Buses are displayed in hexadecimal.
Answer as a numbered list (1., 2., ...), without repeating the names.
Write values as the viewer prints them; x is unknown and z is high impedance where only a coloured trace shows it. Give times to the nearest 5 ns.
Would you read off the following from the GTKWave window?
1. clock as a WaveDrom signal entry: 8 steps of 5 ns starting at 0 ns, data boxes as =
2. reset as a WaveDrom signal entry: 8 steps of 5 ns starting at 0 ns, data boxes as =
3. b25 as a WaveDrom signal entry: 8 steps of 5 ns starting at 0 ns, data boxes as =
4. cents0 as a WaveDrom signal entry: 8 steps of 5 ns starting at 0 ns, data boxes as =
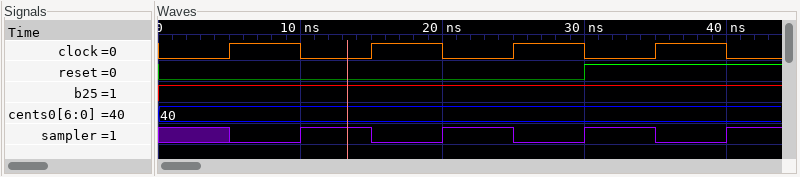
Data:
1. {name: 'clock', wave: '01010101'}
2. {name: 'reset', wave: '0.....1.'}
3. {name: 'b25', wave: '1.......'}
4. {name: 'cents0', wave: '=.......', data: '40'}
